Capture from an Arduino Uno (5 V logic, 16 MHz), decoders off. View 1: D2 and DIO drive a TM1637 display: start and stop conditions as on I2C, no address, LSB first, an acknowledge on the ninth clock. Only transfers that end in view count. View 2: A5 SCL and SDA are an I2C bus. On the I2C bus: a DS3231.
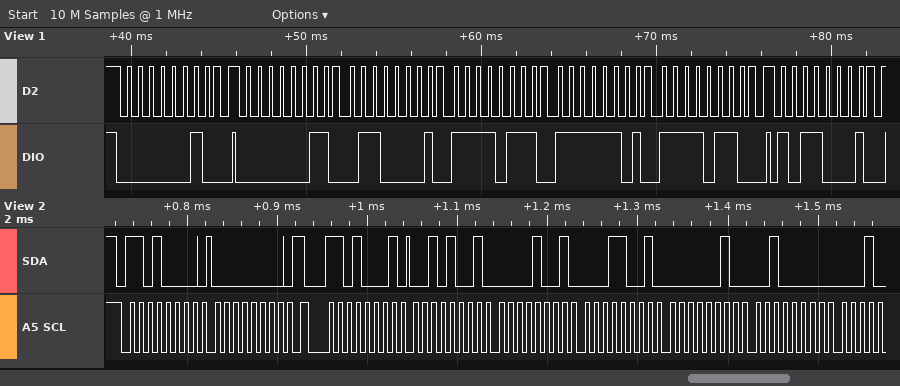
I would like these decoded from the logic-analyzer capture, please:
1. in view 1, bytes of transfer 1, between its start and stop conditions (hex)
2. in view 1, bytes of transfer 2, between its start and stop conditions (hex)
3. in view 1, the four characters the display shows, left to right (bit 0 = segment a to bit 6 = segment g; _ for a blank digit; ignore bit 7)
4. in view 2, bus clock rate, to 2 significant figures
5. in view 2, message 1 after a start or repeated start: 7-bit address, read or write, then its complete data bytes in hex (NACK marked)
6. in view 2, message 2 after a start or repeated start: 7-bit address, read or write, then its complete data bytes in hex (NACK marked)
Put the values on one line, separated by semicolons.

40; C0 86 EF BF 6F; 1909; 100 kHz; 0x68 write: 00; 0x68 read: 29 09 19 02 20
